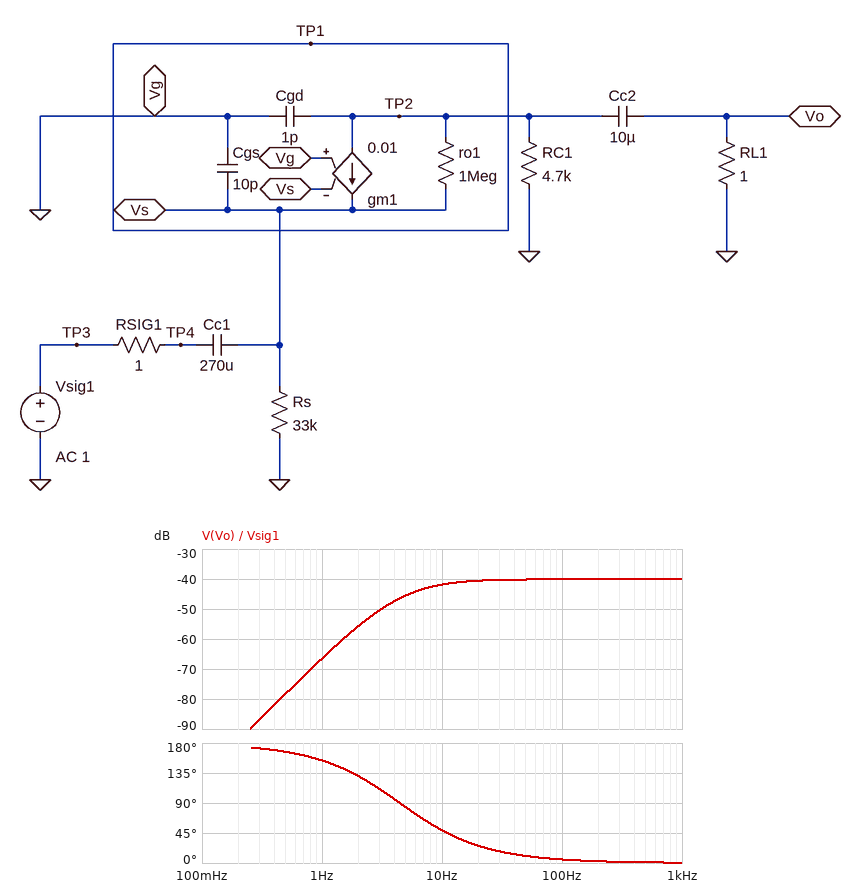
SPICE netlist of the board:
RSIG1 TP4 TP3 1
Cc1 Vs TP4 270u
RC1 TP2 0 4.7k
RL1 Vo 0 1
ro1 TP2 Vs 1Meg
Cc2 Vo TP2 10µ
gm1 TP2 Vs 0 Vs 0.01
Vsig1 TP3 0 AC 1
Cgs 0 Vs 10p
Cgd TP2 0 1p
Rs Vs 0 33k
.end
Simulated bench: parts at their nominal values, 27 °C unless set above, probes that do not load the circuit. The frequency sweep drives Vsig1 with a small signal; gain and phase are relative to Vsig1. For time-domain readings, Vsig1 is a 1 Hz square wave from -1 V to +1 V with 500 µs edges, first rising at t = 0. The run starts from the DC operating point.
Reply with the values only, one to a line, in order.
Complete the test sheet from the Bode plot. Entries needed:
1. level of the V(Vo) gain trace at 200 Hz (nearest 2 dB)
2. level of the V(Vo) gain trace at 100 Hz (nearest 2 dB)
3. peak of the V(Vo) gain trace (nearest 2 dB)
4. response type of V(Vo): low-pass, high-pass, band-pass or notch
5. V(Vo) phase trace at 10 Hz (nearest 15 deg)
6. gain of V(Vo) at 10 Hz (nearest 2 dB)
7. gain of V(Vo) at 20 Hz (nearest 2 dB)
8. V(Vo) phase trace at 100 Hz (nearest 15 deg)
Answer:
-40 dB
-40 dB
-40 dB
high-pass
45 deg
-42 dB
-40 dB
0 deg
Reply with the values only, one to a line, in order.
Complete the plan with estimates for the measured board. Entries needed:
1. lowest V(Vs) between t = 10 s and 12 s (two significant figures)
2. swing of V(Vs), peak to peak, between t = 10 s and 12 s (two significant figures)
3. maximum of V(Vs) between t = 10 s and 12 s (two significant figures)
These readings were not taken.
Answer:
-2.0 V
3.9 V
2.0 V
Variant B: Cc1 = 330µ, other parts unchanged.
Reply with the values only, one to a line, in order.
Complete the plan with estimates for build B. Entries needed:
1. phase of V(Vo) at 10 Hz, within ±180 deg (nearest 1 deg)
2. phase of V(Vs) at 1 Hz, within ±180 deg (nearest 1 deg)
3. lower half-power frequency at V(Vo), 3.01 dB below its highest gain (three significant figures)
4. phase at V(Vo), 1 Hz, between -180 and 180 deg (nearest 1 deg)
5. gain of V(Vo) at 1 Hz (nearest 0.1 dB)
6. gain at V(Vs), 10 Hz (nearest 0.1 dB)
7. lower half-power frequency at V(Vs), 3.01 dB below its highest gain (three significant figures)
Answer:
44 deg
78 deg
6.41 Hz
152 deg
-64.8 dB
-1.0 dB
4.79 Hz
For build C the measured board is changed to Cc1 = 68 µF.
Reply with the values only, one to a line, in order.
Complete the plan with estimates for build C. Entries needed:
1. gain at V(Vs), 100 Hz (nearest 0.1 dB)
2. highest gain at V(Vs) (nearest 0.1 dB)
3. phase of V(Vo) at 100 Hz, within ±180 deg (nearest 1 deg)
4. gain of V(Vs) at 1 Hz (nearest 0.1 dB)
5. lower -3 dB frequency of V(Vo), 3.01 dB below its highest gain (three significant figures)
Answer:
-0.3 dB
-0.1 dB
15 deg
-27.4 dB
23.7 Hz
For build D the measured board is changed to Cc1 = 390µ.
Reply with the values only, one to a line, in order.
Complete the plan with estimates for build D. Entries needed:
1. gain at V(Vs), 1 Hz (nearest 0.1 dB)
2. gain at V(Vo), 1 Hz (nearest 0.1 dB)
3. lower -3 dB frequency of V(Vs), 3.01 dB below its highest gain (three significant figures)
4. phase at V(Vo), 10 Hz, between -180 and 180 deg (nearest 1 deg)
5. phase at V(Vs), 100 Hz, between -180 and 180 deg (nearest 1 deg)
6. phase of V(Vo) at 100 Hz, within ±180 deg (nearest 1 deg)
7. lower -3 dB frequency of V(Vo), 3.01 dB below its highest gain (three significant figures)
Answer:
-12.5 dB
-63.5 dB
4.05 Hz
41 deg
2 deg
4 deg
5.81 Hz
